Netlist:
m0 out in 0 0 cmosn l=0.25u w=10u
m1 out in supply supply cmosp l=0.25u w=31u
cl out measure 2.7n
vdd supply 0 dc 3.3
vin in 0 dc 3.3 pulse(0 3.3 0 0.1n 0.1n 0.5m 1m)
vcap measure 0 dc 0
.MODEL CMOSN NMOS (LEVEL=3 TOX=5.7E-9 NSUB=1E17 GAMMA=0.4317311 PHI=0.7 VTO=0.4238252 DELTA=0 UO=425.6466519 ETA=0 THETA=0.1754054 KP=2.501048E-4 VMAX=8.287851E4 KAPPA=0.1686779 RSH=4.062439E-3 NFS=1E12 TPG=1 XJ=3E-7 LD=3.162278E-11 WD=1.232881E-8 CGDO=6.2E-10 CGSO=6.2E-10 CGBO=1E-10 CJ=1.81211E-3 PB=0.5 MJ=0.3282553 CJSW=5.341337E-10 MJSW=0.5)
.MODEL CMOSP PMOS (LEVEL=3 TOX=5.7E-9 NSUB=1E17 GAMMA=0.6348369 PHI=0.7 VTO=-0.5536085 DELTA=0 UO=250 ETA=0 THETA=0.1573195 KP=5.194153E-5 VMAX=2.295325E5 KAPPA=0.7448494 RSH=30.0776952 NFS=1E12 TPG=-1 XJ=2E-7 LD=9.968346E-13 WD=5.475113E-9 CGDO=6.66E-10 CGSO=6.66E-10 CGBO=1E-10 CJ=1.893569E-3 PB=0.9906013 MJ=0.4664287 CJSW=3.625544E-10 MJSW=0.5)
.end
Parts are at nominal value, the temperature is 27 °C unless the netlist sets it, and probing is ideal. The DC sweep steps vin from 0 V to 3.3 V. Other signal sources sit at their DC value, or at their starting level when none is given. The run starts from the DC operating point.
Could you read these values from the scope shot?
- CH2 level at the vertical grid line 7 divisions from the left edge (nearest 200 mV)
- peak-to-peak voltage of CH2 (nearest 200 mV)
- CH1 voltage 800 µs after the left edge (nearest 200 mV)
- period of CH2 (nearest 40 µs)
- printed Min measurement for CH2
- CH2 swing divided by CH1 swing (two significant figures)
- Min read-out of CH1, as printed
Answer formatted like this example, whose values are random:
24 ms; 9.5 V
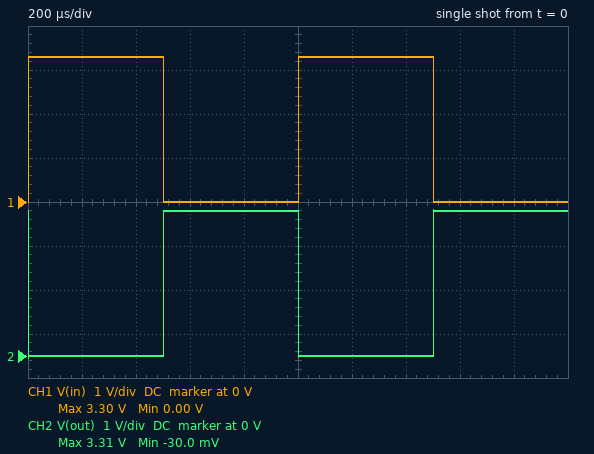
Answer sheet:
0 V; 3.4 V; 0 V; 1.00 ms; -30.0 mV; 1.0; 0.00 V
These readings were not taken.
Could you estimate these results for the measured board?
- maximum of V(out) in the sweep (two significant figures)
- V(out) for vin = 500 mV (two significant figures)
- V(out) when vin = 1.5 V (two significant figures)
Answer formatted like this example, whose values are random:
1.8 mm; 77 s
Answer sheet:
3.3 V; 3.3 V; 2.5 V
